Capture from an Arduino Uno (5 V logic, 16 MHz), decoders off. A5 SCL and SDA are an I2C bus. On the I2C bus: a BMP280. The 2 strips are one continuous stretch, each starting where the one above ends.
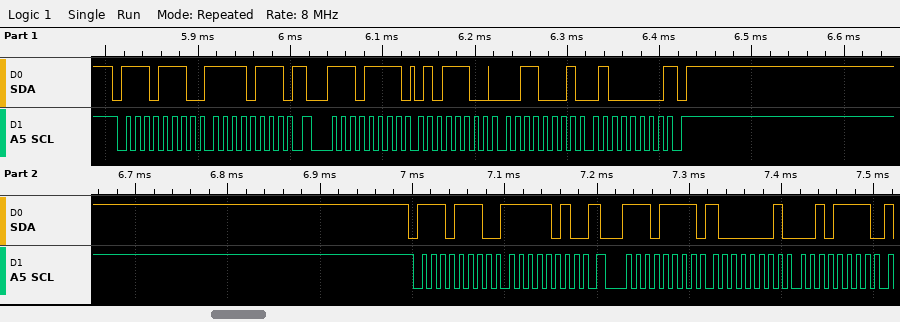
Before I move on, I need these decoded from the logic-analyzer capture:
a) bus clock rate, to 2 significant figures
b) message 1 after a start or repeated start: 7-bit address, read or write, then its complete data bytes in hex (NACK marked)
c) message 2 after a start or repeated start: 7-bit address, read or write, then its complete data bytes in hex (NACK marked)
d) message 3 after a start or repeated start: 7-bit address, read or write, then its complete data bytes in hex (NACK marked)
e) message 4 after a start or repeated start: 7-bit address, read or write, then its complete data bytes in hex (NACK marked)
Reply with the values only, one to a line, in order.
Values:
100 kHz
0x77 write: F7
0x77 read: 5C 31 40 NACK
0x77 write: FA
0x77 read: 81 2F
